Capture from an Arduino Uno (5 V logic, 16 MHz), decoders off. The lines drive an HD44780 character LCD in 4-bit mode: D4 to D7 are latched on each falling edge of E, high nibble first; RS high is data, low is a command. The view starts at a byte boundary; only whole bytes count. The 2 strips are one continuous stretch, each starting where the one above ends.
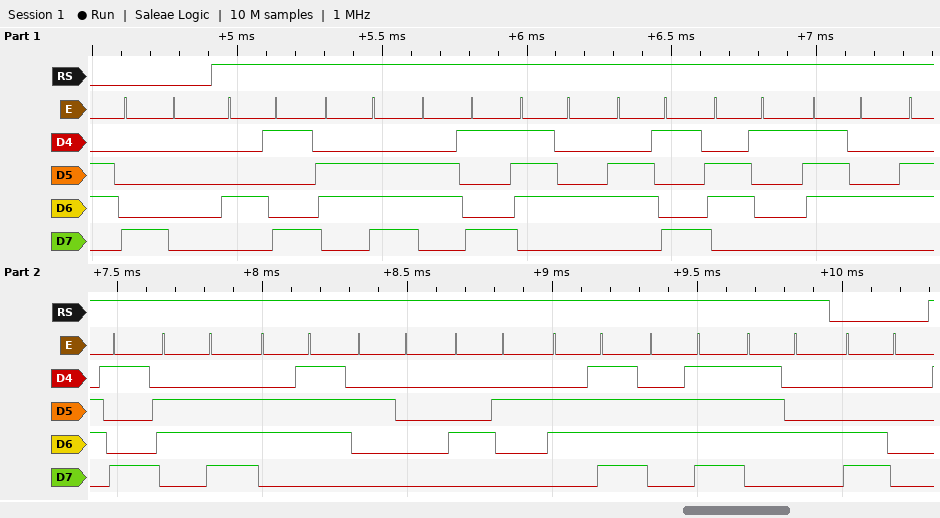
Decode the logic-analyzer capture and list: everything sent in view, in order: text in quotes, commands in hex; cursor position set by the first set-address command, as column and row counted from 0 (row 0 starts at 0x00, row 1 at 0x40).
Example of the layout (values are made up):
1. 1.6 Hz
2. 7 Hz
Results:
1. 0x80 "Initiating Boot" 0xC0
2. column 0, row 0
